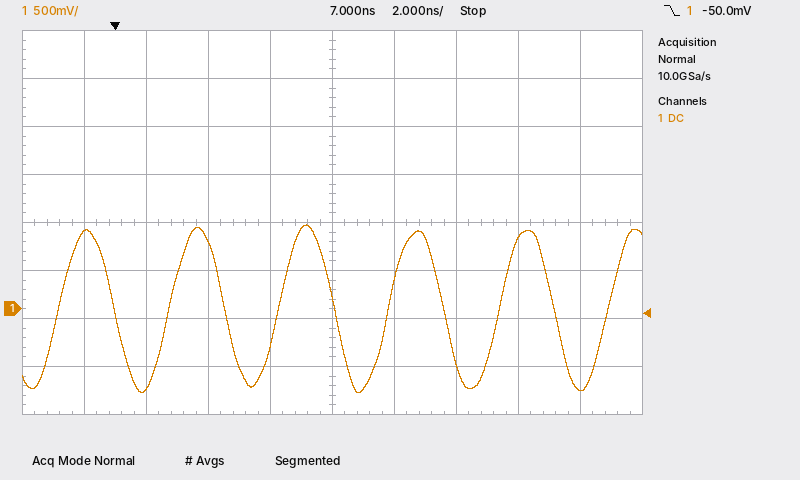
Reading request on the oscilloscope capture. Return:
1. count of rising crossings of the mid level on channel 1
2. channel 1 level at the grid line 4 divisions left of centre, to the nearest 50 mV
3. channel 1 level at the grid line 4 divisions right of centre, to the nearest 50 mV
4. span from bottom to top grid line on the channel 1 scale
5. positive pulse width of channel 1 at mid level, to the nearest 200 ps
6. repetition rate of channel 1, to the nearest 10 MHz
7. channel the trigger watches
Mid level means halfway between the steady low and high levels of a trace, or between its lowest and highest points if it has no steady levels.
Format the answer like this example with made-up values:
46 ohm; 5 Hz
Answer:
6; 800 mV; -850 mV; 4 V; 1.8 ns; 280 MHz; channel 1
